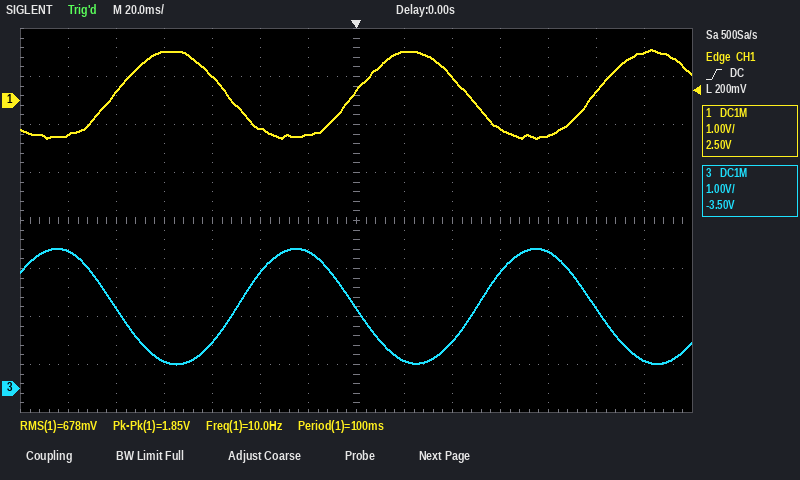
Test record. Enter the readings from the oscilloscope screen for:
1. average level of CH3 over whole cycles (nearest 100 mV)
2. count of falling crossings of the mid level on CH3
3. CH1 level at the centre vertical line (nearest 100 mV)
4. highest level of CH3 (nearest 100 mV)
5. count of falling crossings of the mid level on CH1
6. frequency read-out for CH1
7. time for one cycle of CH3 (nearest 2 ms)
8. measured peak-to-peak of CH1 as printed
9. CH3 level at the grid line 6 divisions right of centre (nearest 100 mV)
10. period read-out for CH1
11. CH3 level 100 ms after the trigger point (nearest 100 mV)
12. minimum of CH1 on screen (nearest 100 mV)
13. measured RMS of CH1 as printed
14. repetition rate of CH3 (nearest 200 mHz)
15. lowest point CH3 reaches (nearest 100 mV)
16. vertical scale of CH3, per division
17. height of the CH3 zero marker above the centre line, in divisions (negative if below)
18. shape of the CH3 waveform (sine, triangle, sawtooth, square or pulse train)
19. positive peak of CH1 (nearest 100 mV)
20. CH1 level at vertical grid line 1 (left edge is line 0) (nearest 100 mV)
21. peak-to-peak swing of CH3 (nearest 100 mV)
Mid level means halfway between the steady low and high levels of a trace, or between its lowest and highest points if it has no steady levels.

1.7 V
3
200 mV
2.9 V
2
10.0 Hz
100 ms
1.85 V
600 mV
100 ms
1.7 V
-800 mV
678 mV
10.0 Hz
500 mV
1 V
-3.5 div
sine
1.1 V
-700 mV
2.4 V
